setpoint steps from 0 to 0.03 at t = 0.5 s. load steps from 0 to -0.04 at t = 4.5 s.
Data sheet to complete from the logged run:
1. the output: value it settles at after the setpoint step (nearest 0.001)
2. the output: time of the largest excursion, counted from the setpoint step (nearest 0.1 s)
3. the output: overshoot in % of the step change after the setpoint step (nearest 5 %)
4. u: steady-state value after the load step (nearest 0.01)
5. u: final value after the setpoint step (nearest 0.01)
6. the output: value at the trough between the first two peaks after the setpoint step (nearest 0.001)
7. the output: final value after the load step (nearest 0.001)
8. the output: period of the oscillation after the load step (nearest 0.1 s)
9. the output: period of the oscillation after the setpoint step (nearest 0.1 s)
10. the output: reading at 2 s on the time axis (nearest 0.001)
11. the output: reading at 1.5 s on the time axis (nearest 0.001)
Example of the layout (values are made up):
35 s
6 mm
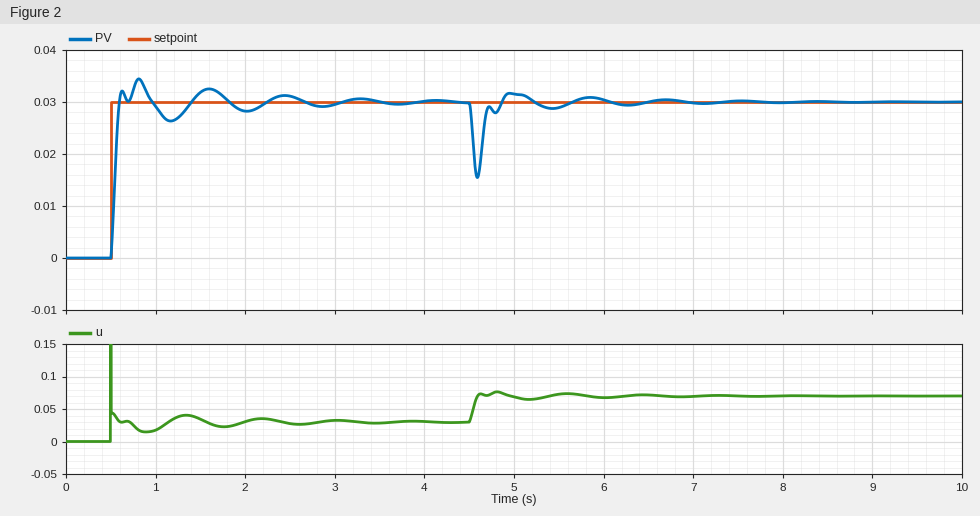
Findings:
0.030
0.3 s
15 %
0.07
0.03
0.026
0.030
0.8 s
0.8 s
0.028
0.032
